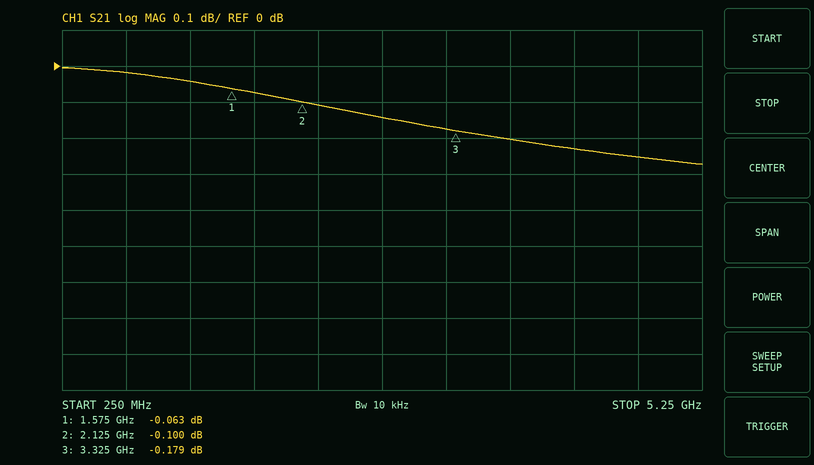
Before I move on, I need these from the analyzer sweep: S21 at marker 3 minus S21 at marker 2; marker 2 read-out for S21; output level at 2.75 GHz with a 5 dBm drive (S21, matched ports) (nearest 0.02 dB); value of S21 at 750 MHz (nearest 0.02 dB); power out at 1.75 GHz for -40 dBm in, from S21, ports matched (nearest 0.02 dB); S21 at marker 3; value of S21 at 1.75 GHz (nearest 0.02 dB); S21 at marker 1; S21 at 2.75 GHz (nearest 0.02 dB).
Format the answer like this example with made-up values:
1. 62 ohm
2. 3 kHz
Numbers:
1. -0.079 dB
2. -0.100 dB
3. 4.86 dBm
4. -0.02 dB
5. -40.08 dBm
6. -0.179 dB
7. -0.08 dB
8. -0.063 dB
9. -0.14 dB
